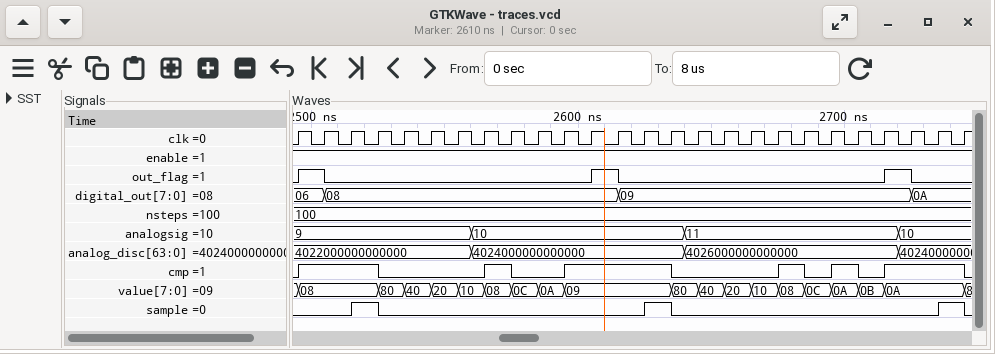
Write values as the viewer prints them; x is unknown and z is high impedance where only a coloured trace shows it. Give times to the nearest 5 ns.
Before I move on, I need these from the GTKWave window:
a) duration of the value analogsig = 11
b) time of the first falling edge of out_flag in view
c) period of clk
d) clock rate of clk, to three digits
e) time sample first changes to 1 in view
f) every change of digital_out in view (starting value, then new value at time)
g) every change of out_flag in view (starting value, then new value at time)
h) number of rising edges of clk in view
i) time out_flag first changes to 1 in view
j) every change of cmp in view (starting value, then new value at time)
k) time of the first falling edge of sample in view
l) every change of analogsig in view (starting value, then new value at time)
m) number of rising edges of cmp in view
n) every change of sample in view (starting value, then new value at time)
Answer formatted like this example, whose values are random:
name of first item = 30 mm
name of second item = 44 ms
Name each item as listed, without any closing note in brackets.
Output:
duration of the value analogsig = 11 = 80 ns
time of the first falling edge of out_flag in view = 2505 ns
period of clk = 10 ns
clock rate of clk, to three digits = 100 MHz
time sample first changes to 1 in view = 2515 ns
every change of digital_out in view = 06, 08 at 2505 ns, 09 at 2615 ns, 0A at 2725 ns
every change of out_flag in view = 0, 1 at 2495 ns, 0 at 2505 ns, 1 at 2605 ns, 0 at 2615 ns, 1 at 2715 ns, 0 at 2725 ns
number of rising edges of clk in view = 26
time out_flag first changes to 1 in view = 2495 ns
every change of cmp in view = 0, 1 at 2495 ns, 0 at 2525 ns, 1 at 2565 ns, 0 at 2575 ns, 1 at 2595 ns, 0 at 2635 ns, 1 at 2675 ns, 0 at 2685 ns, 1 at 2695 ns, 0 at 2705 ns, 1 at 2715 ns, 0 at 2745 ns
time of the first falling edge of sample in view = 2525 ns
every change of analogsig in view = 9, 10 at 2560 ns, 11 at 2640 ns, 10 at 2720 ns
number of rising edges of cmp in view = 6
every change of sample in view = 0, 1 at 2515 ns, 0 at 2525 ns, 1 at 2625 ns, 0 at 2635 ns, 1 at 2735 ns, 0 at 2745 ns
